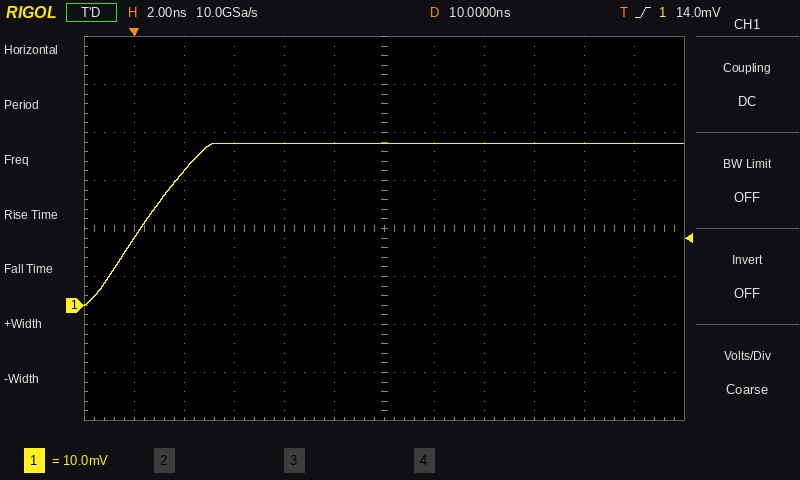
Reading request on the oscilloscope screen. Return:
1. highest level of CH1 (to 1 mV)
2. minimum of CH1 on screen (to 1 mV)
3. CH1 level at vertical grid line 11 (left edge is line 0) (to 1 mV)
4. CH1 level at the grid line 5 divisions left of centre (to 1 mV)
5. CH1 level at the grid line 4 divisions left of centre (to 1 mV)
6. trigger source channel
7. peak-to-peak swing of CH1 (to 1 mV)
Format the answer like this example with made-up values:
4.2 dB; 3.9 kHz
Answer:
34 mV; 0 mV; 34 mV; 14 mV; 28 mV; CH1; 34 mV
